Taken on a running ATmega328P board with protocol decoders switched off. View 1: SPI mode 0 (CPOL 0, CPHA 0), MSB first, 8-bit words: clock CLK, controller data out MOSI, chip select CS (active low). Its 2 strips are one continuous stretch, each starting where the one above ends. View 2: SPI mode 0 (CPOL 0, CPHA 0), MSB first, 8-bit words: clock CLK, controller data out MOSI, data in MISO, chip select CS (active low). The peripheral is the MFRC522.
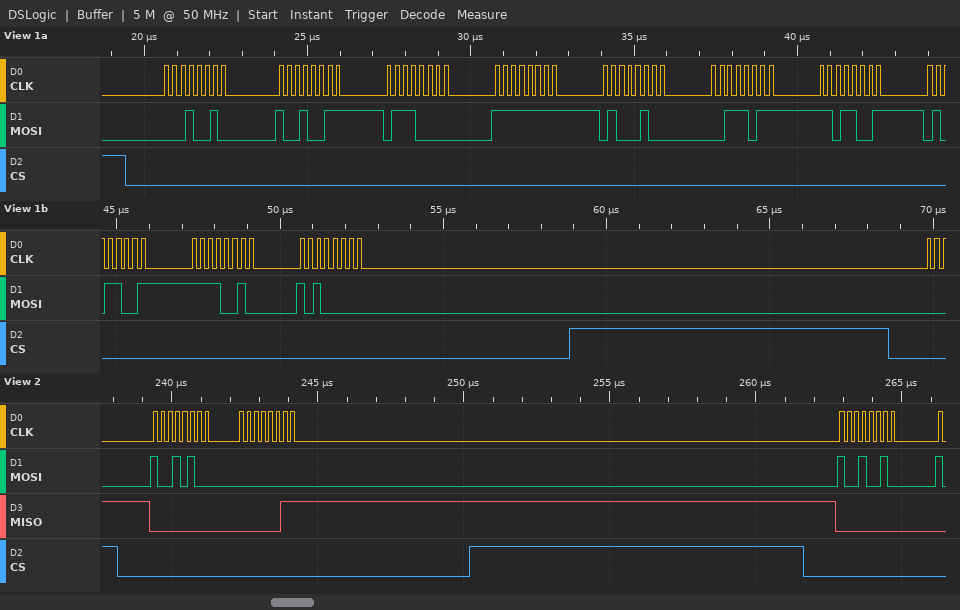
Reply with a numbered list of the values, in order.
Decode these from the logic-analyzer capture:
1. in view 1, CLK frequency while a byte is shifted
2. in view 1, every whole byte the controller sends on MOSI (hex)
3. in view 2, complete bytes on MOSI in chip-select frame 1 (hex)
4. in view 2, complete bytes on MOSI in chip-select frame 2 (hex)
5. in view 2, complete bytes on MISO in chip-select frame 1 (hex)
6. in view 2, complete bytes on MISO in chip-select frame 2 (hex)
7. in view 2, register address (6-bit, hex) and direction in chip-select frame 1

1. 4 MHz
2. 12 93 70 FF 44 3B D9 59 F2 A0
3. 94 00
4. 92
5. 00 03
6. 00
7. 0x0A read
